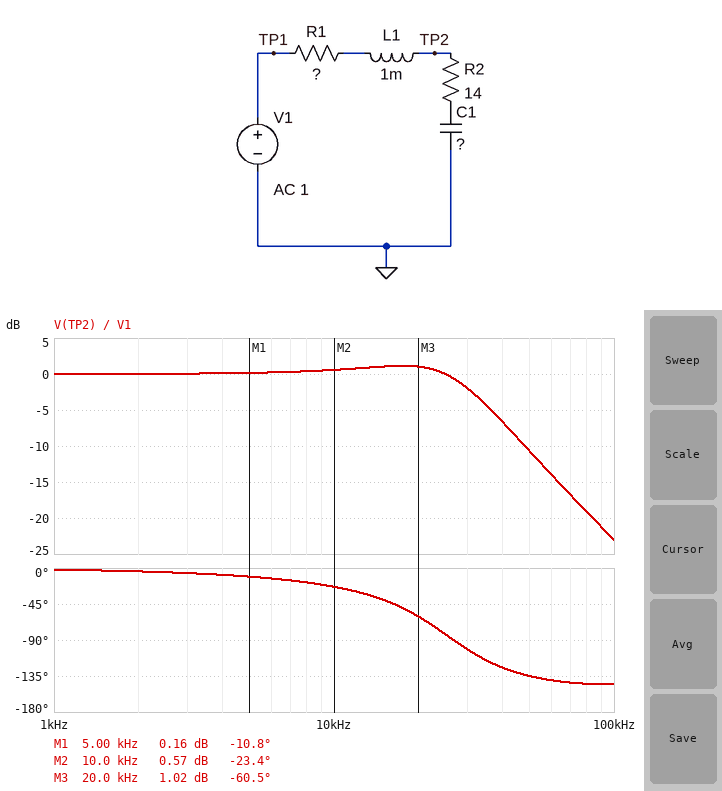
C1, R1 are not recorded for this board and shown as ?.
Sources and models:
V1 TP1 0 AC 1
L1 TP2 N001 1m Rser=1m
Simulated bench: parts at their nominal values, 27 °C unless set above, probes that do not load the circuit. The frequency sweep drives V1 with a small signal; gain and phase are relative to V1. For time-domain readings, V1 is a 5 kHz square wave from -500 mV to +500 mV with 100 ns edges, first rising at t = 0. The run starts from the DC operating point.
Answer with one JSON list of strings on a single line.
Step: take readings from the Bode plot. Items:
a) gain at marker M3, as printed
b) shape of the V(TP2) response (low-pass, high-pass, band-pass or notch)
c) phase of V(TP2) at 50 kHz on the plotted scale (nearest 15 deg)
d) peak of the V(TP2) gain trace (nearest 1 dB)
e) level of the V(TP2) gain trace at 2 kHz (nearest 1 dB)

["1.02 dB", "low-pass", "-135 deg", "1 dB", "0 dB"]
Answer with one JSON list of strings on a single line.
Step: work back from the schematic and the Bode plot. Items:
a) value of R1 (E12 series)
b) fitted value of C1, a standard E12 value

["150 Ω", "39 nF"]
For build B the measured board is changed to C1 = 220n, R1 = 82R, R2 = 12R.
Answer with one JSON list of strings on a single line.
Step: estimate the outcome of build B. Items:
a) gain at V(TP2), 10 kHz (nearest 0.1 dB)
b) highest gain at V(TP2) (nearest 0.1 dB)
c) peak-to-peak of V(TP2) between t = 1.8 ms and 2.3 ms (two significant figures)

["-2.2 dB", "0 dB", "1.1 V"]
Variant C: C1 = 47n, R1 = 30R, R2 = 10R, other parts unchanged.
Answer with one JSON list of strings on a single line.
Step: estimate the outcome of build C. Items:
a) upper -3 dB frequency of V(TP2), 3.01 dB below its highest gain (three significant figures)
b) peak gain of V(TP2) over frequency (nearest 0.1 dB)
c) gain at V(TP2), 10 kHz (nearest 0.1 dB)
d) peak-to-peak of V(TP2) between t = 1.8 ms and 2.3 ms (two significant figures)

["25.8 kHz", "11.3 dB", "1.7 dB", "2.3 V"]
